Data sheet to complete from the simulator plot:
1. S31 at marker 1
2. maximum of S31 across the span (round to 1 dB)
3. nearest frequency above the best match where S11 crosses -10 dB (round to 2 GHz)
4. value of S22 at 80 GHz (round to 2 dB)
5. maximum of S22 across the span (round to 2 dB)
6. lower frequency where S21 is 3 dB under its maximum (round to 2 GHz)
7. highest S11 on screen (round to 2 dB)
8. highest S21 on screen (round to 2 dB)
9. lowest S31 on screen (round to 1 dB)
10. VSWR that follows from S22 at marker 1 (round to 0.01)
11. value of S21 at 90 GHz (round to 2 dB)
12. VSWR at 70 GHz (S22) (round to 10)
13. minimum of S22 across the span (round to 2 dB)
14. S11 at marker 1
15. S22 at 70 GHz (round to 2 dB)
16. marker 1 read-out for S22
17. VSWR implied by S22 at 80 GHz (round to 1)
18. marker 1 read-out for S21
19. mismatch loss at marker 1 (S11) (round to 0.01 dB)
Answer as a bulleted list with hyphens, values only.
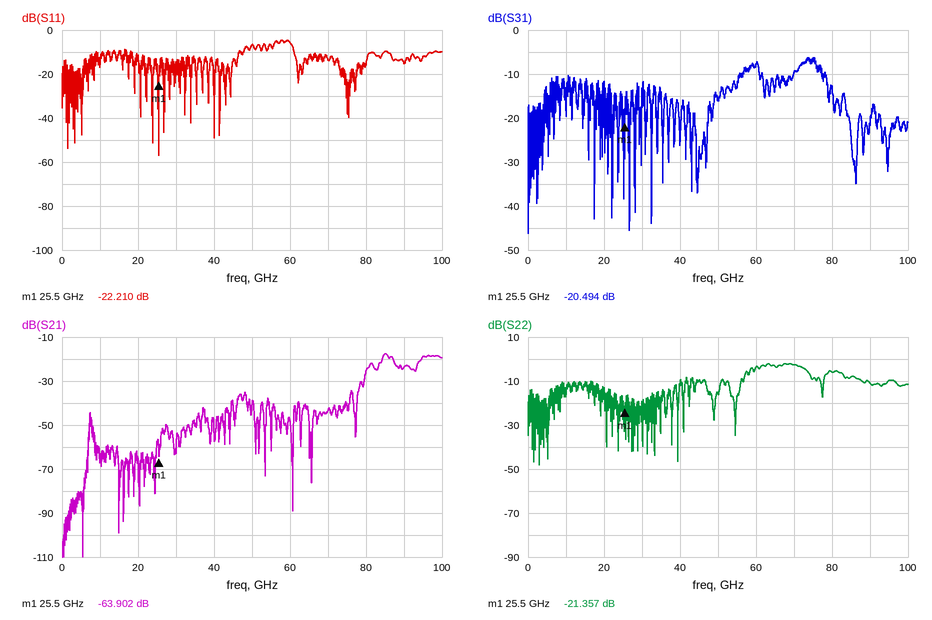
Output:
- -20.494 dB
- -6 dB
- 46 GHz
- -6 dB
- -2 dB
- 84 GHz
- -4 dB
- -18 dB
- -46 dB
- 1.19
- -24 dB
- 10
- -48 dB
- -22.210 dB
- -2 dB
- -21.357 dB
- 3
- -63.902 dB
- 0.03 dB
